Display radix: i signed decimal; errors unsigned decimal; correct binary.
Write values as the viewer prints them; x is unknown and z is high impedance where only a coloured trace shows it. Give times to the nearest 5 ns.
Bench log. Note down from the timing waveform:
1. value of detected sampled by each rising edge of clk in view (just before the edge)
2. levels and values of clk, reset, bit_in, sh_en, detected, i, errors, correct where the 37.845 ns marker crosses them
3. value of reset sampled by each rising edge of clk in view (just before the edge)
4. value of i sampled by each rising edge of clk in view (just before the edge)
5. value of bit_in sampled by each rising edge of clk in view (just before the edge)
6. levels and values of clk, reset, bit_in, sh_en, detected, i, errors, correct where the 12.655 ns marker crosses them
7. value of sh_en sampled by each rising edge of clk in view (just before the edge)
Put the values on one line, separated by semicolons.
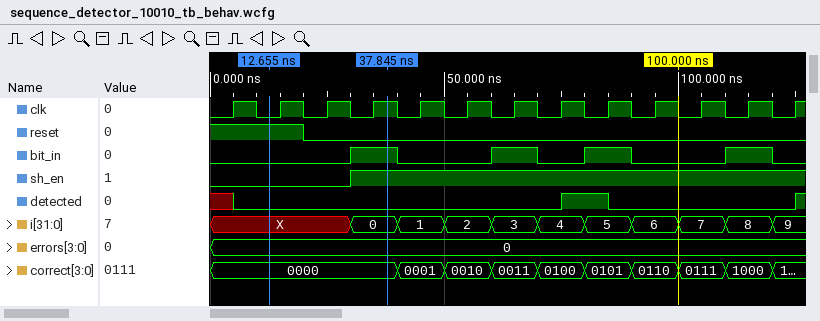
x 0 0 0 0 0 0 0 1 0 0 0 0; clk=1, reset=0, bit_in=1, sh_en=1, detected=0, i=0, errors=0, correct=0000; 1 1 0 0 0 0 0 0 0 0 0 0 0; X, X, X, 0, 1, 2, 3, 4, 5, 6, 7, 8, 9; 0 0 0 1 0 0 1 0 1 0 0 1 0; clk=0, reset=1, bit_in=0, sh_en=0, detected=0, i=X, errors=0, correct=0000; 0 0 0 1 1 1 1 1 1 1 1 1 1
